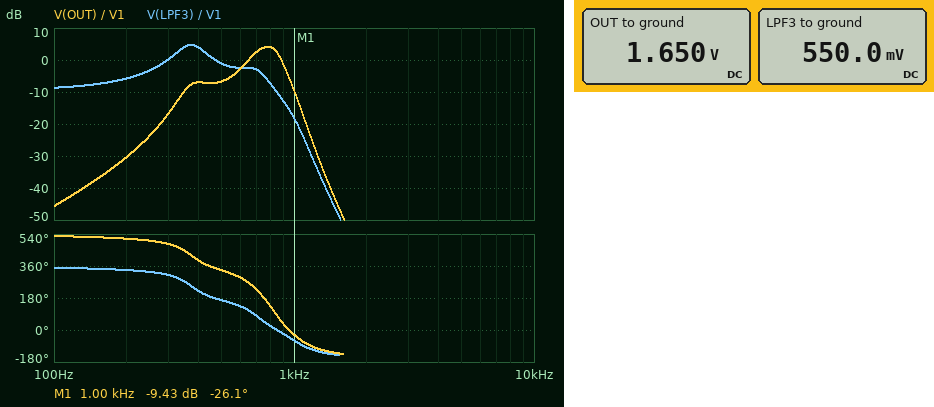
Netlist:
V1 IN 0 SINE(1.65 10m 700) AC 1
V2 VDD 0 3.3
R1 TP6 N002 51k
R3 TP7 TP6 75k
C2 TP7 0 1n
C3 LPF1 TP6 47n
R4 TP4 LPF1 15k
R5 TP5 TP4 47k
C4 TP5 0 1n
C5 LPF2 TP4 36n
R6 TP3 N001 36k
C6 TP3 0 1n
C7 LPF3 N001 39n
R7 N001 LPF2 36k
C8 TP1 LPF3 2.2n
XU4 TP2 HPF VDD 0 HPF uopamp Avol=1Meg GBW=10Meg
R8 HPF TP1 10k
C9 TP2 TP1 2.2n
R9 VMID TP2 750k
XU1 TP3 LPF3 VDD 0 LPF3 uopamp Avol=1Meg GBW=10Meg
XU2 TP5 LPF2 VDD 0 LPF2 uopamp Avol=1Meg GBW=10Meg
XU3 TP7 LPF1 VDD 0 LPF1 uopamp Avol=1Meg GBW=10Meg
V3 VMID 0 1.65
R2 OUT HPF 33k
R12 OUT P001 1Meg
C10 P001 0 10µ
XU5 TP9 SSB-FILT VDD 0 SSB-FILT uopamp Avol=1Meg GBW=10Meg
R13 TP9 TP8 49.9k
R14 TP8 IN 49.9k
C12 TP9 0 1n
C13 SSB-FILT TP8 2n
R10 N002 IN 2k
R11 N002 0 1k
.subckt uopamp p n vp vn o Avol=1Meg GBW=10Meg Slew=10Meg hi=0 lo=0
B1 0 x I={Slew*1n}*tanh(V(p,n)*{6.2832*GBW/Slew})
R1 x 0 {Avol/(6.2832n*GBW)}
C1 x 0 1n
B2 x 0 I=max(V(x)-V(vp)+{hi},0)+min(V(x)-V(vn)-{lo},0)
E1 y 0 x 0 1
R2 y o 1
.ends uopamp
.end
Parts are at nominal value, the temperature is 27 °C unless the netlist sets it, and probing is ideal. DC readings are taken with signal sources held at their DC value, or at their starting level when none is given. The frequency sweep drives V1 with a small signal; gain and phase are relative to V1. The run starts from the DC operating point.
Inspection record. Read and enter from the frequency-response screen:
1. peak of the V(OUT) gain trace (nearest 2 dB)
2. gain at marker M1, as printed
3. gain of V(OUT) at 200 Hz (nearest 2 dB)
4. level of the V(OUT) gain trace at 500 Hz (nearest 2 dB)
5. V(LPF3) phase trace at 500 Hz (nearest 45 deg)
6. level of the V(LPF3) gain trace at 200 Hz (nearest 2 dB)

4 dB
-9.43 dB
-30 dB
-6 dB
180 deg
-6 dB
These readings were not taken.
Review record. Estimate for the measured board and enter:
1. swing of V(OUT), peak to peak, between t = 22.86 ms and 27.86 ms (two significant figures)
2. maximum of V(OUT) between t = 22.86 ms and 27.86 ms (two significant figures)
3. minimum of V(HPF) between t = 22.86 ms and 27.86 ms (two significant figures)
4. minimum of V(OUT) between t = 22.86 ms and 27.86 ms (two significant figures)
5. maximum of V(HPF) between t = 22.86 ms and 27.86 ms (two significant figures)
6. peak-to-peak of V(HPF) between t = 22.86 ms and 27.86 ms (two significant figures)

27 mV
1.7 V
1.6 V
1.6 V
1.7 V
28 mV
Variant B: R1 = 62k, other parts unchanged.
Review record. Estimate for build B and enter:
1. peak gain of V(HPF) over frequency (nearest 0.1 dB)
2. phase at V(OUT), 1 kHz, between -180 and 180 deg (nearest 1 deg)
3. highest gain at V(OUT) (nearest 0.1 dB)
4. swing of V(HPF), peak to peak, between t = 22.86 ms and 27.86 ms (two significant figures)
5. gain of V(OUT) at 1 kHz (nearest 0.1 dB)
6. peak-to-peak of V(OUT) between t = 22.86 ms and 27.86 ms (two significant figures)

2.3 dB
-27 deg
2.0 dB
22 mV
-11.3 dB
21 mV
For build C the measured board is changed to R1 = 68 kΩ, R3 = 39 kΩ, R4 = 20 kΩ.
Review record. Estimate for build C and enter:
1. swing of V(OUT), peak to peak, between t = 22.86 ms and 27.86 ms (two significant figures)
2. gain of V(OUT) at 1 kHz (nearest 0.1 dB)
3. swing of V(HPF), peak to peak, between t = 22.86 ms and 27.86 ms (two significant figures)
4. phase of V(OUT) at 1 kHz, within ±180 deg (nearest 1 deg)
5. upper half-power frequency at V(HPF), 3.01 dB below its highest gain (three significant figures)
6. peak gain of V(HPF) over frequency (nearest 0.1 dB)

59 mV
-8.4 dB
61 mV
-62 deg
853 Hz
11.0 dB
